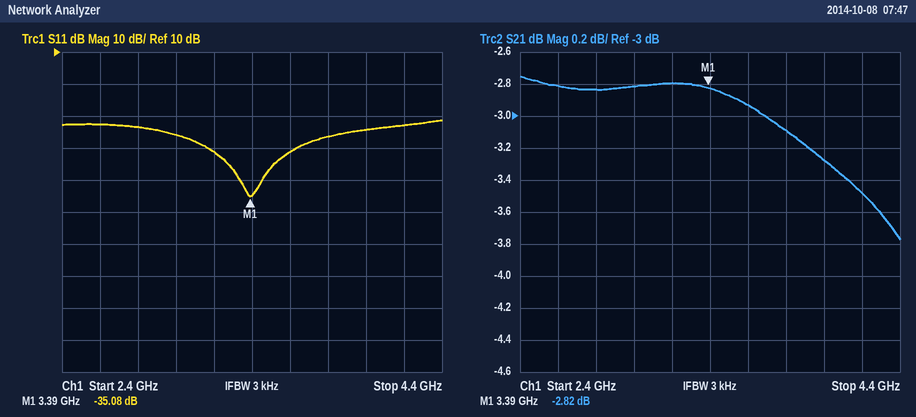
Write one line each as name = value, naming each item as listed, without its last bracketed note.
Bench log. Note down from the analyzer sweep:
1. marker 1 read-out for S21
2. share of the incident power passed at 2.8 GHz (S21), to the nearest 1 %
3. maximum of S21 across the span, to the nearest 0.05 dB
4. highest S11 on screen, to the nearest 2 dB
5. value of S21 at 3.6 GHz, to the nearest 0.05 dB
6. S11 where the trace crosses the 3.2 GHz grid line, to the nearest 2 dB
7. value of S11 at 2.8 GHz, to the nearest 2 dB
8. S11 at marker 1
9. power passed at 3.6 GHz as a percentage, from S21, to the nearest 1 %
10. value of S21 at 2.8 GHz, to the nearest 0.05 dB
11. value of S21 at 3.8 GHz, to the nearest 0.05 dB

marker 1 read-out for S21 = -2.82 dB
share of the incident power passed at 2.8 GHz (S21), to the nearest 1 % = 52 %
maximum of S21 across the span, to the nearest 0.05 dB = -2.75 dB
highest S11 on screen, to the nearest 2 dB = -12 dB
value of S21 at 3.6 GHz, to the nearest 0.05 dB = -2.95 dB
S11 where the trace crosses the 3.2 GHz grid line, to the nearest 2 dB = -22 dB
value of S11 at 2.8 GHz, to the nearest 2 dB = -14 dB
S11 at marker 1 = -35.08 dB
power passed at 3.6 GHz as a percentage, from S21, to the nearest 1 % = 51 %
value of S21 at 2.8 GHz, to the nearest 0.05 dB = -2.85 dB
value of S21 at 3.8 GHz, to the nearest 0.05 dB = -3.10 dB
